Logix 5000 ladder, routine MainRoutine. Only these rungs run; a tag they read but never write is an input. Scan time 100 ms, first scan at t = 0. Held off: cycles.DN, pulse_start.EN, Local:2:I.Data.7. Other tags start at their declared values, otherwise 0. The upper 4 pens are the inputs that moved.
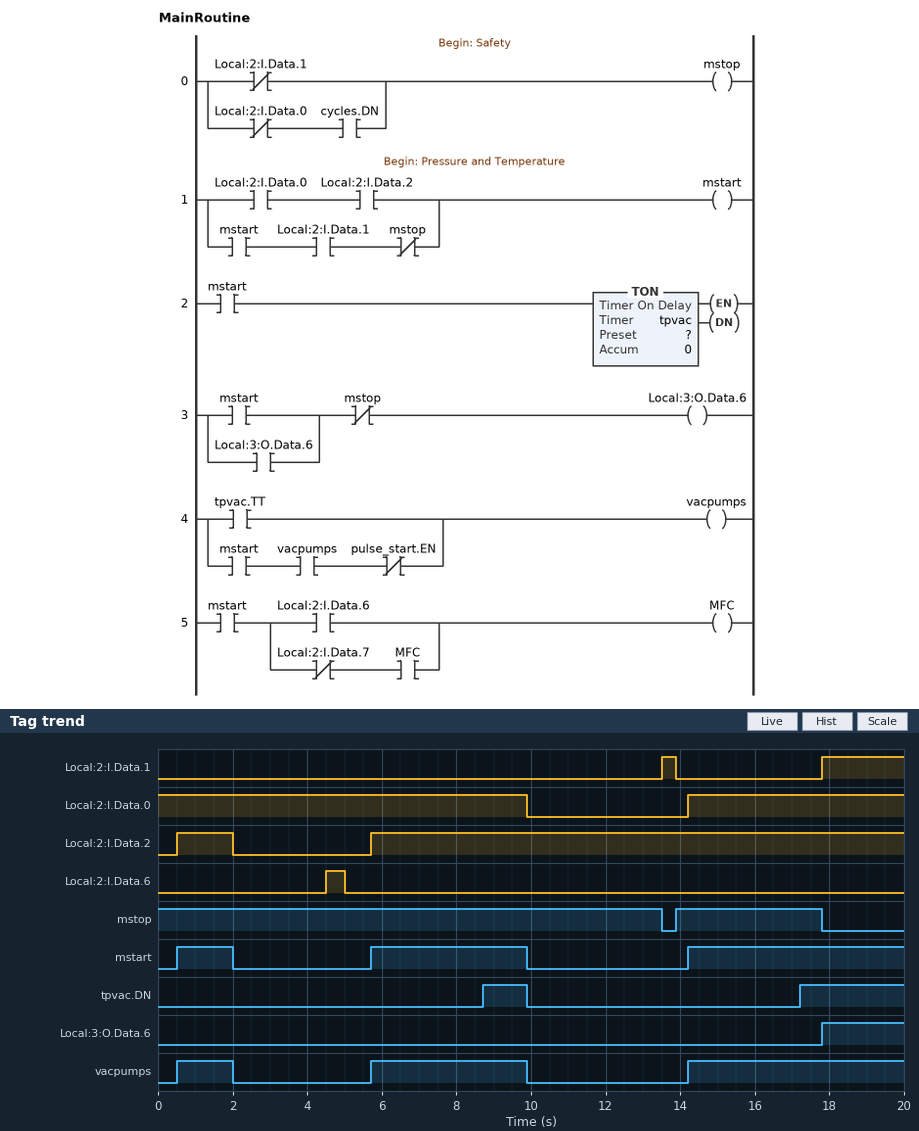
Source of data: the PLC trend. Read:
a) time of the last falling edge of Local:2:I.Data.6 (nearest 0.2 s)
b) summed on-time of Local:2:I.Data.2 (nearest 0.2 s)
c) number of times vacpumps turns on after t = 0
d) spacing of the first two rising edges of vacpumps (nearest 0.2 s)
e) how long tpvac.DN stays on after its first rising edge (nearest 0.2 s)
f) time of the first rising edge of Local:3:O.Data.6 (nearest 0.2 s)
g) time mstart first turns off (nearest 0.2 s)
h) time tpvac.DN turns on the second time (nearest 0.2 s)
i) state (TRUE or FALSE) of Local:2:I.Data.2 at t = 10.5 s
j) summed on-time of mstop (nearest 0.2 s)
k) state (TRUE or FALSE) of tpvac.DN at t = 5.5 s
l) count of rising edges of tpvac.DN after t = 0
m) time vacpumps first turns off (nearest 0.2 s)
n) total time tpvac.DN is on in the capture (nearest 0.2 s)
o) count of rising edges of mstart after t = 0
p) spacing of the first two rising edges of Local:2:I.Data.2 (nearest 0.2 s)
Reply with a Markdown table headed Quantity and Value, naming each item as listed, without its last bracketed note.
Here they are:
| Quantity | Value |
|---|---|
| time of the last falling edge of Local:2:I.Data.6 | 5.0 s |
| summed on-time of Local:2:I.Data.2 | 15.8 s |
| number of times vacpumps turns on after t = 0 | 3 |
| spacing of the first two rising edges of vacpumps | 5.2 s |
| how long tpvac.DN stays on after its first rising edge | 1.2 s |
| time of the first rising edge of Local:3:O.Data.6 | 17.8 s |
| time mstart first turns off | 2.0 s |
| time tpvac.DN turns on the second time | 17.2 s |
| state (TRUE or FALSE) of Local:2:I.Data.2 at t = 10.5 s | TRUE |
| summed on-time of mstop | 17.4 s |
| state (TRUE or FALSE) of tpvac.DN at t = 5.5 s | FALSE |
| count of rising edges of tpvac.DN after t = 0 | 2 |
| time vacpumps first turns off | 2.0 s |
| total time tpvac.DN is on in the capture | 4.0 s |
| count of rising edges of mstart after t = 0 | 3 |
| spacing of the first two rising edges of Local:2:I.Data.2 | 5.2 s |
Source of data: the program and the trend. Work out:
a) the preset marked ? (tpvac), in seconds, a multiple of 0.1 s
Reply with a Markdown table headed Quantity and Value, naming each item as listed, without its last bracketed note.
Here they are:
| Quantity | Value |
|---|---|
| the preset marked ? (tpvac), in seconds, a multiple of 0.1 s | 3.0 s |
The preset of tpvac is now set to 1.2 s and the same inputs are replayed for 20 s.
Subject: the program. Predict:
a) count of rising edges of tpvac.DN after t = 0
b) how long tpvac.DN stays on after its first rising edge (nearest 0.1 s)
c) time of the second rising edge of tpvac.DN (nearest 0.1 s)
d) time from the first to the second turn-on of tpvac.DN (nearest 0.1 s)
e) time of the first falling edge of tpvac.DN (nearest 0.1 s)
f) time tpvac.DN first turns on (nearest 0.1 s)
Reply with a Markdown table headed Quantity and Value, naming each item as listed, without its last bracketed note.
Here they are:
| Quantity | Value |
|---|---|
| count of rising edges of tpvac.DN after t = 0 | 3 |
| how long tpvac.DN stays on after its first rising edge | 0.3 s |
| time of the second rising edge of tpvac.DN | 6.9 s |
| time from the first to the second turn-on of tpvac.DN | 5.2 s |
| time of the first falling edge of tpvac.DN | 2.0 s |
| time tpvac.DN first turns on | 1.7 s |
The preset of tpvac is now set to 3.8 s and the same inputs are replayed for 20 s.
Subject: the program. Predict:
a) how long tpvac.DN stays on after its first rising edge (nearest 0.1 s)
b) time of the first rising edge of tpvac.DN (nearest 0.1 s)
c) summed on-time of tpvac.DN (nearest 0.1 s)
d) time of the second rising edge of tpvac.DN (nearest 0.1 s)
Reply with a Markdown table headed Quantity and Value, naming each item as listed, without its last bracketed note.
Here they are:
| Quantity | Value |
|---|---|
| how long tpvac.DN stays on after its first rising edge | 0.4 s |
| time of the first rising edge of tpvac.DN | 9.5 s |
| summed on-time of tpvac.DN | 2.4 s |
| time of the second rising edge of tpvac.DN | 18.0 s |
